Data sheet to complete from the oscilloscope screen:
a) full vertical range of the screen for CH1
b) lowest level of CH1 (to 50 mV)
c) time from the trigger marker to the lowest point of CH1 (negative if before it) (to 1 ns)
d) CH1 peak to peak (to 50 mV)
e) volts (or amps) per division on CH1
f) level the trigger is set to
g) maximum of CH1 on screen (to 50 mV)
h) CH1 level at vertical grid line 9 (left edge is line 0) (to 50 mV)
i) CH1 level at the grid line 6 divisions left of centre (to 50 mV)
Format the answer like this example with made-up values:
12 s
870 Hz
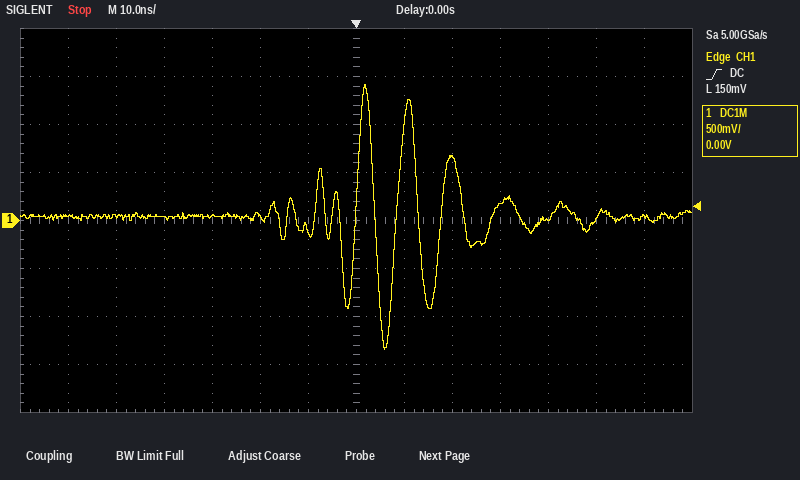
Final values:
4 V
-1.35 V
+6 ns
2.75 V
500 mV
150 mV
1.40 V
650 mV
50 mV
